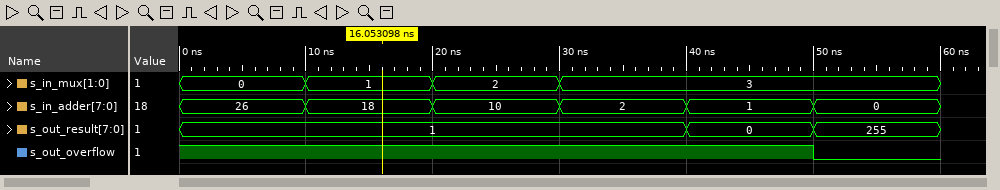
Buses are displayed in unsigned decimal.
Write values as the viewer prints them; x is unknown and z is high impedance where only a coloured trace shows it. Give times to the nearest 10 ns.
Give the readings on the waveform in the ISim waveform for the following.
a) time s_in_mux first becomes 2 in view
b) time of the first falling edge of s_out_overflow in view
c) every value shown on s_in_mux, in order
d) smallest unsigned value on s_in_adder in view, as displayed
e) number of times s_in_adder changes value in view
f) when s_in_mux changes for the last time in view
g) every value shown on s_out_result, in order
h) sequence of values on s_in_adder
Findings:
20 ns
50 ns
0, 1, 2, 3
0
5
30 ns
1, 0, 255
26, 18, 10, 2, 1, 0
